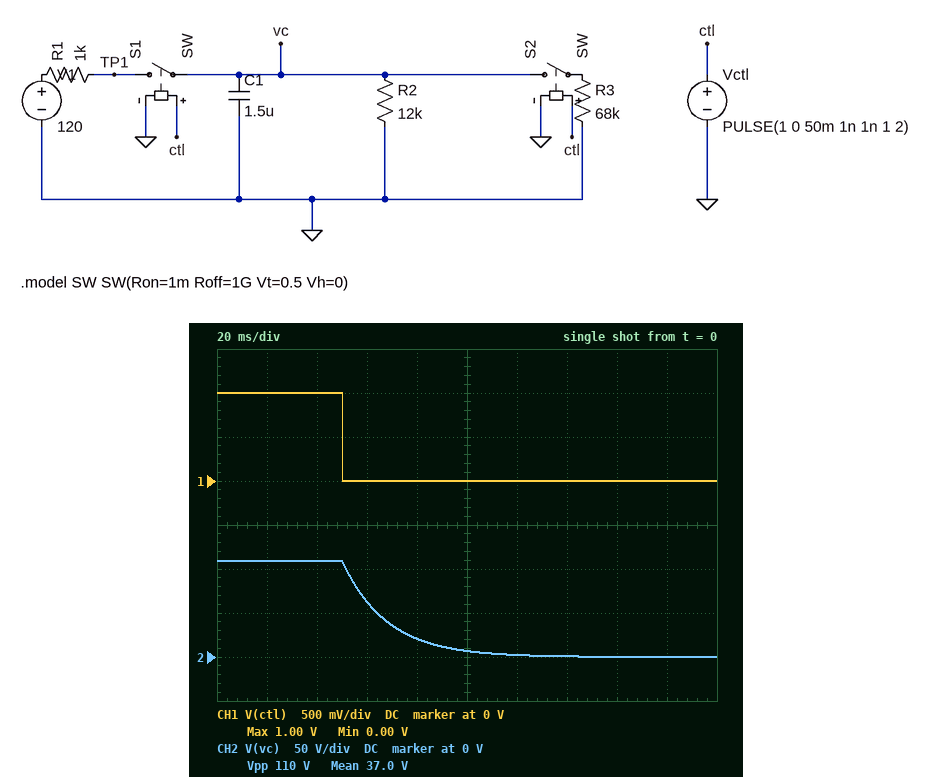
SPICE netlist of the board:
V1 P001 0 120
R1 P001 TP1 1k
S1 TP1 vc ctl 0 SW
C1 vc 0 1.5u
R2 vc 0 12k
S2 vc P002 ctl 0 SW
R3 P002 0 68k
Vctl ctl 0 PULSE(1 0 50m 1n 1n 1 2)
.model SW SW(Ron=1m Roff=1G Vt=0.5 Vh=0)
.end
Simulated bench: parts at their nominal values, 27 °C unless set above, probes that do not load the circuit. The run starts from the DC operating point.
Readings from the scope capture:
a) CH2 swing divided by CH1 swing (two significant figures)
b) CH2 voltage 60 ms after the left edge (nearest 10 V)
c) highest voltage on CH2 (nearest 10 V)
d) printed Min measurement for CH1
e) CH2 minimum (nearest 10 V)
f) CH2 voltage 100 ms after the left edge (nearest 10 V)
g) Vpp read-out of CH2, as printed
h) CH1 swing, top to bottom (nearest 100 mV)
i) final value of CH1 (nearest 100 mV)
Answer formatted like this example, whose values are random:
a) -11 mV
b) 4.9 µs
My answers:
a) 110
b) 60 V
c) 110 V
d) 0.00 V
e) 0 V
f) 10 V
g) 110 V
h) 1.0 V
i) 0 V
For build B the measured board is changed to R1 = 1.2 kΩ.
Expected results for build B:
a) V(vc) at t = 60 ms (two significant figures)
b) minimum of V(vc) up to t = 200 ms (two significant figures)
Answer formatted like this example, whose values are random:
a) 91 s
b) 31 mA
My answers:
a) 62 V
b) 27 mV
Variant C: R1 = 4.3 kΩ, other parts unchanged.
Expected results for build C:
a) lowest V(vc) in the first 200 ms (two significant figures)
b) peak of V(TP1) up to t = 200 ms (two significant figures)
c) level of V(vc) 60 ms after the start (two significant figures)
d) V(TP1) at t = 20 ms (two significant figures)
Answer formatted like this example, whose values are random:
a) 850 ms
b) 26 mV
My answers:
a) 22 mV
b) 120 V
c) 48 V
d) 84 V
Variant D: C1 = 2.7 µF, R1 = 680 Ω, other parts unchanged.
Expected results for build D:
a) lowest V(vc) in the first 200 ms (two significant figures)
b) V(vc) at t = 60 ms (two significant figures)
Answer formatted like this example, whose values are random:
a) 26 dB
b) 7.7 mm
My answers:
a) 1.1 V
b) 83 V
